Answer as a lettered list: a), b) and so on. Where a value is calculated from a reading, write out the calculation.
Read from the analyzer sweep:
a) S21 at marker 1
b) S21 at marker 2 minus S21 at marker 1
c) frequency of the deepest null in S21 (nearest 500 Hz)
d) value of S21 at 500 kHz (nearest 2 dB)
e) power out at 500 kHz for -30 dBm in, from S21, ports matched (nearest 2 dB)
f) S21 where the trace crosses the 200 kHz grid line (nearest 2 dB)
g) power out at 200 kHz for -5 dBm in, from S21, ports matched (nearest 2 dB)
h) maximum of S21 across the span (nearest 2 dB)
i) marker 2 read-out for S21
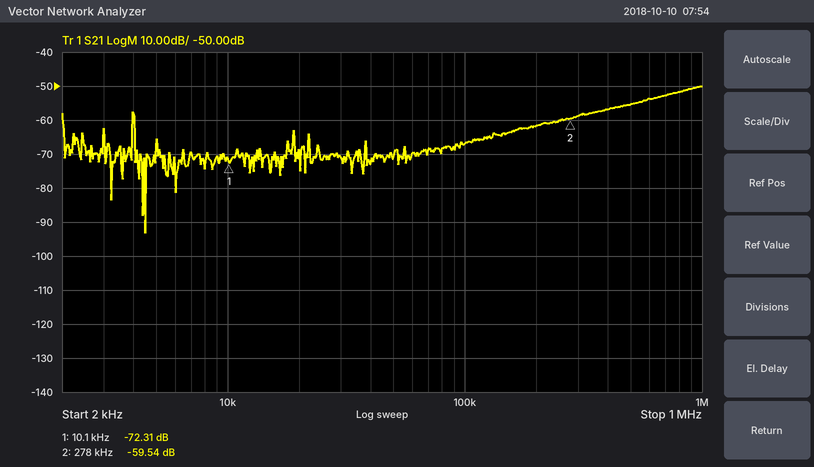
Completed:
a) -72.31 dB
b) -59.54 − (-72.31) = 12.77 dB
c) 4.5 kHz
d) -56 dB
e) -30 dBm + (-56 dB) = -86 dBm
f) -62 dB
g) -5 dBm + (-62 dB) = -66 dBm
h) -50 dB
i) -59.54 dB
